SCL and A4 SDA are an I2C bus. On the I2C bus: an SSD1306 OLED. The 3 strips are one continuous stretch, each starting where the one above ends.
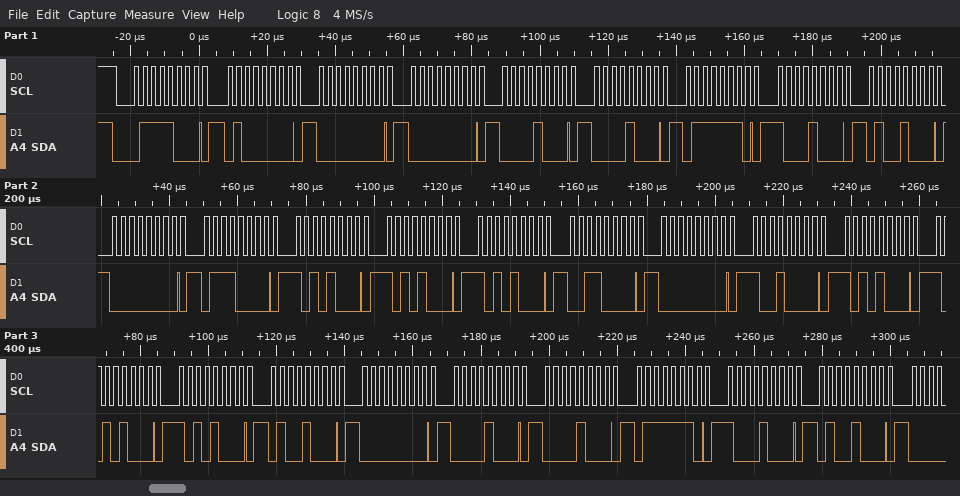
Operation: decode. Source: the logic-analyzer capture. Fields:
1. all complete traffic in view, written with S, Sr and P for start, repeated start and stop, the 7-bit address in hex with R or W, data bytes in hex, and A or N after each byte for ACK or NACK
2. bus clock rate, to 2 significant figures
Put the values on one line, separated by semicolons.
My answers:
S 3CW A 40 A 00 A 00 A 08 A 08 A 7E A 88 A 48 A 00 A 70 A A8 A A8 A A8 A 30 A 00 A 90 A A8 A A8 A A8 A 48 A 00 A 08 A 08 A 7E A 88 A 48 A; 400 kHz
